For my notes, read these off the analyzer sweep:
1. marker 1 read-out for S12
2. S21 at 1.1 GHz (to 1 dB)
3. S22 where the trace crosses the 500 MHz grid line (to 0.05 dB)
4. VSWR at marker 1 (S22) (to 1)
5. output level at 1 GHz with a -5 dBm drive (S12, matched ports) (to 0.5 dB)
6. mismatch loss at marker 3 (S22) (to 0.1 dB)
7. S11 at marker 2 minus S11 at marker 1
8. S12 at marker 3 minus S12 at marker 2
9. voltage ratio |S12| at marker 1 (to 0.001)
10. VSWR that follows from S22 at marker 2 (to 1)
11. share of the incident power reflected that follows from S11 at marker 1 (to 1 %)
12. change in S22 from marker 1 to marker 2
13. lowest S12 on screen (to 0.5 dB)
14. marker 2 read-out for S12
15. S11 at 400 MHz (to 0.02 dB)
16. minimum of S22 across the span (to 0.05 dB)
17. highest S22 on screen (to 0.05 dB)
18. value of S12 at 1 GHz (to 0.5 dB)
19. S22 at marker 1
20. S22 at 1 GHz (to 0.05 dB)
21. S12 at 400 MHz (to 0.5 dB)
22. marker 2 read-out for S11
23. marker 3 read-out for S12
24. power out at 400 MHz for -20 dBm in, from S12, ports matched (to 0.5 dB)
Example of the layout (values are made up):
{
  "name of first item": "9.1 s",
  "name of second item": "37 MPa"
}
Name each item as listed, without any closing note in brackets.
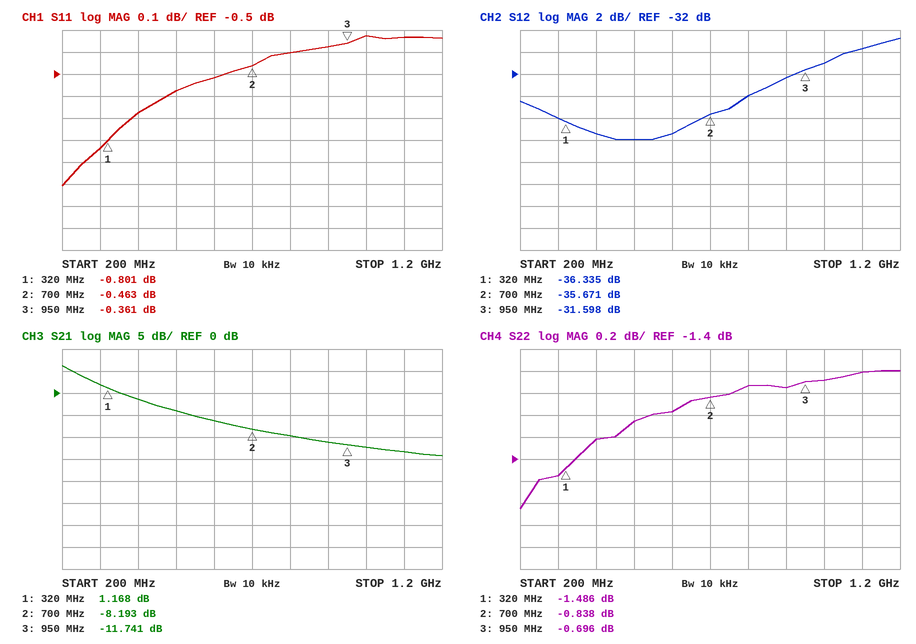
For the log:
{
  "marker 1 read-out for S12": "-36.335 dB",
  "S21 at 1.1 GHz": "-13 dB",
  "S22 where the trace crosses the 500 MHz grid line": "-1.05 dB",
  "VSWR at marker 1 (S22)": "12",
  "output level at 1 GHz with a -5 dBm drive (S12, matched ports)": "-36.0 dBm",
  "mismatch loss at marker 3 (S22)": "8.3 dB",
  "S11 at marker 2 minus S11 at marker 1": "0.338 dB",
  "S12 at marker 3 minus S12 at marker 2": "4.073 dB",
  "voltage ratio |S12| at marker 1": "0.015",
  "VSWR that follows from S22 at marker 2": "21",
  "share of the incident power reflected that follows from S11 at marker 1": "83 %",
  "change in S22 from marker 1 to marker 2": "0.648 dB",
  "lowest S12 on screen": "-38.0 dB",
  "marker 2 read-out for S12": "-35.671 dB",
  "S11 at 400 MHz": "-0.68 dB",
  "minimum of S22 across the span": "-1.85 dB",
  "highest S22 on screen": "-0.60 dB",
  "value of S12 at 1 GHz": "-31.0 dB",
  "S22 at marker 1": "-1.486 dB",
  "S22 at 1 GHz": "-0.70 dB",
  "S12 at 400 MHz": "-37.5 dB",
  "marker 2 read-out for S11": "-0.463 dB",
  "marker 3 read-out for S12": "-31.598 dB",
  "power out at 400 MHz for -20 dBm in, from S12, ports matched": "-57.5 dBm"
}
